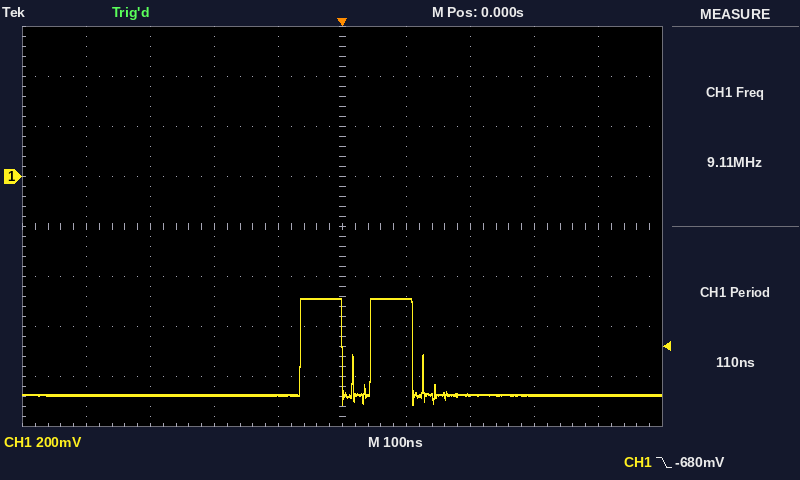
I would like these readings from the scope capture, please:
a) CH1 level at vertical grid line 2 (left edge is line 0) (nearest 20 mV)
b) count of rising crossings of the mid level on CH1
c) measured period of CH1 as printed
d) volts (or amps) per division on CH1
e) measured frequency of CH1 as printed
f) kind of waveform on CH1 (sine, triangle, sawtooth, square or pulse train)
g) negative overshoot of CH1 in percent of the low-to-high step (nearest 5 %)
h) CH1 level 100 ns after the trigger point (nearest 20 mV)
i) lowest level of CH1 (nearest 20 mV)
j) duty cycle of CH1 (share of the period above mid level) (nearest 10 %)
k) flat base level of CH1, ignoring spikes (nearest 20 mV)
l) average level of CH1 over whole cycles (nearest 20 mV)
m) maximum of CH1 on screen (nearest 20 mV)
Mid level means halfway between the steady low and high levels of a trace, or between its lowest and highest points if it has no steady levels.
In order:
-880 mV
2
110 ns
200 mV
9.11 MHz
pulse train
10 %
-480 mV
-920 mV
60 %
-880 mV
-640 mV
-480 mV
